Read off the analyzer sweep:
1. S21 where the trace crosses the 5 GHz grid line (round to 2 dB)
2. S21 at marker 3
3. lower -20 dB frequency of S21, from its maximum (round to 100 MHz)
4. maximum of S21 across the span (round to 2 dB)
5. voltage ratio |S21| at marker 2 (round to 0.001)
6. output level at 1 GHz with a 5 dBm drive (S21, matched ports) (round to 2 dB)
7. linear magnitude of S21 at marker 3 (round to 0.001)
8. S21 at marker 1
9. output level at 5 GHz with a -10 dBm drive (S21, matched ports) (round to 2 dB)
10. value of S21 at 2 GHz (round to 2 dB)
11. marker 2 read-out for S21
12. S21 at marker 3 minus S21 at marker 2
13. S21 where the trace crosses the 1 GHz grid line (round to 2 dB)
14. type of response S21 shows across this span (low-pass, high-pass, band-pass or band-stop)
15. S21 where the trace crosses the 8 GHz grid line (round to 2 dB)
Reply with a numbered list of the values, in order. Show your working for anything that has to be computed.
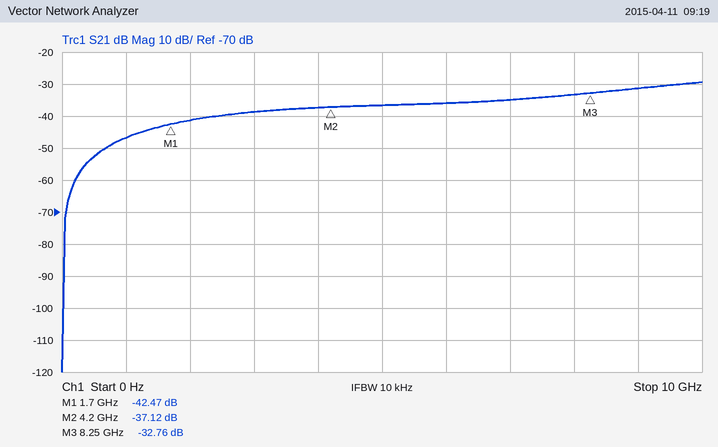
1. -36 dB
2. -32.76 dB
3. 700 MHz
4. -30 dB
5. 10^(-37.12/20) ≈ 0.014
6. 5 dBm + (-46 dB) = -42 dBm
7. 10^(-32.76/20) ≈ 0.023
8. -42.47 dB
9. -10 dBm + (-36 dB) = -46 dBm
10. -42 dB
11. -37.12 dB
12. -32.76 − (-37.12) = 4.36 dB
13. -46 dB
14. high-pass
15. -34 dB
